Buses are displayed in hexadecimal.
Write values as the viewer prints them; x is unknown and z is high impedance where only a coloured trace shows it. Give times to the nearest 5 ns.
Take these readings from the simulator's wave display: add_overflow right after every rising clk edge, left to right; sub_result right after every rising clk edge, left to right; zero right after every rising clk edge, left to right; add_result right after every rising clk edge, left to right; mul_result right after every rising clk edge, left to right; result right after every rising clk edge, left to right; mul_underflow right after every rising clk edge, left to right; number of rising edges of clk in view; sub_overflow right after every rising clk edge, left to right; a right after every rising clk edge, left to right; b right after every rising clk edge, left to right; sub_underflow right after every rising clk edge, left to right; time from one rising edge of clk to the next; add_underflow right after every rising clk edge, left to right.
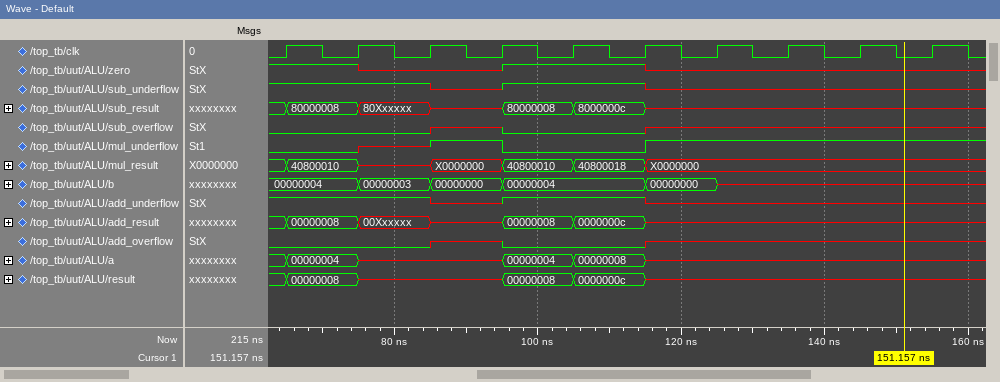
0 0 x 0 0 x x x x x
80000008, 80Xxxxxx, x, 80000008, 8000000c, x, x, x, x, x
1 x x 1 1 x x x x x
00000008, 00Xxxxxx, x, 00000008, 0000000c, x, x, x, x, x
40800010, x, X0000000, 40800010, 40800018, X0000000, X0000000, X0000000, X0000000, X0000000
00000008, x, x, 00000008, 0000000c, x, x, x, x, x
0 x 1 0 0 1 1 1 1 1
10
0 0 x 0 0 x x x x x
00000004, x, x, 00000004, 00000008, x, x, x, x, x
00000004, 00000003, 00000000, 00000004, 00000004, 00000000, x, x, x, x
1 1 x 1 1 x x x x x
10 ns
1 1 x 1 1 x x x x x
